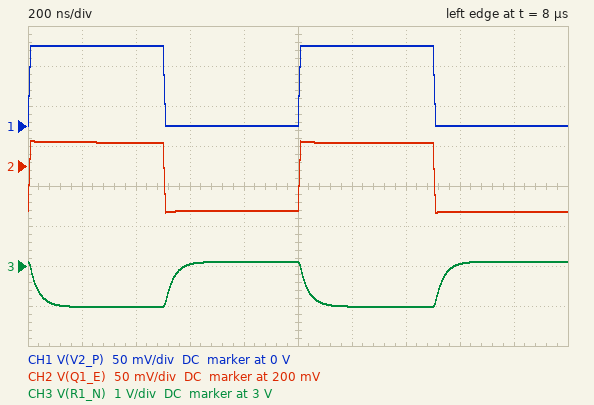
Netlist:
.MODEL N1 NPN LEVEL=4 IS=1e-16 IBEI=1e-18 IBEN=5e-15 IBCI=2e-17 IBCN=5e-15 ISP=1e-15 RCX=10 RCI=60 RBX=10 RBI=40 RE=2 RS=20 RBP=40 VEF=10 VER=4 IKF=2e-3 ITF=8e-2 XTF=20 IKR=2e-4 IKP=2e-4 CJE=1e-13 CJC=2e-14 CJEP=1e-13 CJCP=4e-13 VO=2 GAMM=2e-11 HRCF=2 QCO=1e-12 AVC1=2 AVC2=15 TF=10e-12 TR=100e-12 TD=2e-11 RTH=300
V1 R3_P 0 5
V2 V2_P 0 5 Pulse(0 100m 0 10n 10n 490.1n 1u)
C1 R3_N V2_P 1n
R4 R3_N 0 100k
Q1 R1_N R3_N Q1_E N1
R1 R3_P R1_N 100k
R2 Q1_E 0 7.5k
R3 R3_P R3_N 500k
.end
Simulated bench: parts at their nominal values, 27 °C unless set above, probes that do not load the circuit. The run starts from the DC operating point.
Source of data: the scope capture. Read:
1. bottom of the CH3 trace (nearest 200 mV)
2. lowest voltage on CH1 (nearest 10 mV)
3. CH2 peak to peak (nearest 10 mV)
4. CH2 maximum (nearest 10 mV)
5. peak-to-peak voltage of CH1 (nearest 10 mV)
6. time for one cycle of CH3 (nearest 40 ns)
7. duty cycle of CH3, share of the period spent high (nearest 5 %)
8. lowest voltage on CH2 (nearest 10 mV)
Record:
2.0 V
0 V
90 mV
230 mV
100 mV
1.00 µs
50 %
140 mV
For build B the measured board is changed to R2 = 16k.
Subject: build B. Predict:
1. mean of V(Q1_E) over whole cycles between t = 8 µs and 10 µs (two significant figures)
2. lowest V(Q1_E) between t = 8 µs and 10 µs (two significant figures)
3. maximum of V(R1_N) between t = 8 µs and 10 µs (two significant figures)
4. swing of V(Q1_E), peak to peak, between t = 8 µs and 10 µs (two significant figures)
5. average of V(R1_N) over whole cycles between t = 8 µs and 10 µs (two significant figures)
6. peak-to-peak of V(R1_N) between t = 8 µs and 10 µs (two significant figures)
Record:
220 mV
170 mV
3.9 V
91 mV
3.6 V
540 mV
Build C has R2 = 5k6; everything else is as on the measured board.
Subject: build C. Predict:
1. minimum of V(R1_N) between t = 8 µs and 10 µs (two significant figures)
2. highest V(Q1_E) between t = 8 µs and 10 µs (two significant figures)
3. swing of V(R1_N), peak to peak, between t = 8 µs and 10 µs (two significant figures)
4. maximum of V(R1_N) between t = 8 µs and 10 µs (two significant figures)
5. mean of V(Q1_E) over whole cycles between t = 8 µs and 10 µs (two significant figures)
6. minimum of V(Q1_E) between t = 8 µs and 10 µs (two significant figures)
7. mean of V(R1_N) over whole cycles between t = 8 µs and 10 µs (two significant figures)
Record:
1.2 V
220 mV
1.5 V
2.7 V
170 mV
130 mV
2.0 V
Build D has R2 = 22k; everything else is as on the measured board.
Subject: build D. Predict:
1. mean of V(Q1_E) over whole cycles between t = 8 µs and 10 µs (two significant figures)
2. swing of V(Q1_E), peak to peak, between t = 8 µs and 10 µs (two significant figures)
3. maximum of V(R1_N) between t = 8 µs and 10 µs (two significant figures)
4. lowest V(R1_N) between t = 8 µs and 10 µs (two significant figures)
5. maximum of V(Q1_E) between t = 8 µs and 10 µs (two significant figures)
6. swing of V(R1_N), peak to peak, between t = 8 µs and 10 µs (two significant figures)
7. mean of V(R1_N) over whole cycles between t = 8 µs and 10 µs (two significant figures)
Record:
230 mV
92 mV
4.1 V
3.7 V
280 mV
400 mV
3.9 V
